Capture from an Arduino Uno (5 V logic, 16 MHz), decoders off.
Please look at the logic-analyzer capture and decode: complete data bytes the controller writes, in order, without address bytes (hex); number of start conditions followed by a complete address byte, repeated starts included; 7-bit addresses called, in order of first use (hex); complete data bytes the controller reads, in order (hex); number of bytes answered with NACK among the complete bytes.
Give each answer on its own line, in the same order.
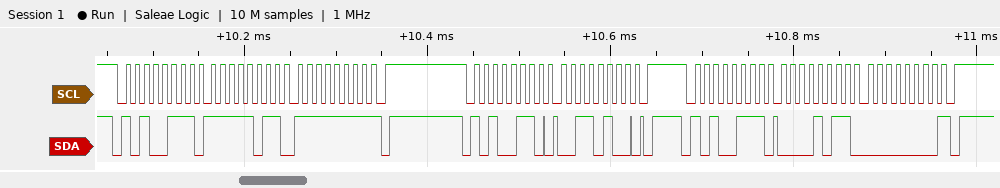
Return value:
34
3
0x53
FB FF 0B 00
2
